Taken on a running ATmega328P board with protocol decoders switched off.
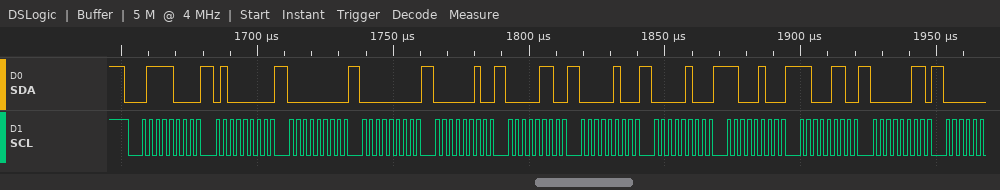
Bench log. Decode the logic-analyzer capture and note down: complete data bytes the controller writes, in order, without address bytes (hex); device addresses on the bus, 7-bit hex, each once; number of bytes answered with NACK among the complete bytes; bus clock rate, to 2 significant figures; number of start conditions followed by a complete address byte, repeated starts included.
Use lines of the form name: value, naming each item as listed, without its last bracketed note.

complete data bytes the controller writes, in order, without address bytes: 40 00 00 02 06 04 04 C4 C6 03
device addresses on the bus, 7-bit hex, each once: 0x3C
number of bytes answered with NACK among the complete bytes: 0
bus clock rate, to 2 significant figures: 400 kHz
number of start conditions followed by a complete address byte, repeated starts included: 1
